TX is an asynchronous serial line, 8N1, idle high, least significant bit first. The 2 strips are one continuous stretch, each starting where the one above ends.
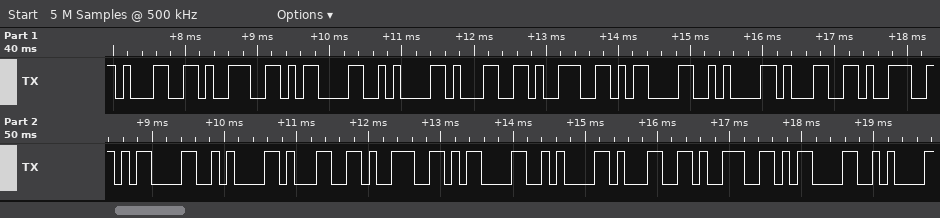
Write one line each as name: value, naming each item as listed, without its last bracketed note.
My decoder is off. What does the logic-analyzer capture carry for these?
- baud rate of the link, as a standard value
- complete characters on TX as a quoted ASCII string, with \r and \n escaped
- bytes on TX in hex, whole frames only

baud rate of the link, as a standard value: 9600 baud
complete characters on TX as a quoted ASCII string, with \r and \n escaped: "19\r\n19\r\n19\r\n19\r\n19\r\n"
bytes on TX in hex, whole frames only: 31 39 0D 0A 31 39 0D 0A 31 39 0D 0A 31 39 0D 0A 31 39 0D 0A
